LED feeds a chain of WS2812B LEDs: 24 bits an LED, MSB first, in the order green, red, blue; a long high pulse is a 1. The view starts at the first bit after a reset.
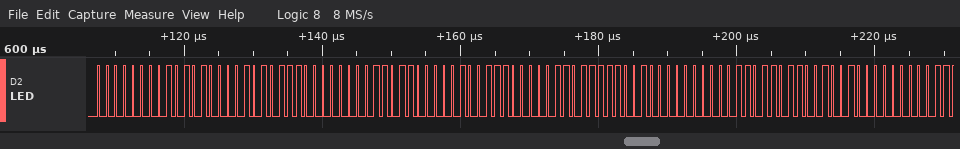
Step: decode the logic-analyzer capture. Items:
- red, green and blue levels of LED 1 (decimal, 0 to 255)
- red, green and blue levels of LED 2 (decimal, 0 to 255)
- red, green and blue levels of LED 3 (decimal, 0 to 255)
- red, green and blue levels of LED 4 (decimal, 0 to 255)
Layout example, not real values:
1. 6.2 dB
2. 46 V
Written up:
1. 168, 0, 87
2. 216, 0, 39
3. 249, 6, 0
4. 201, 54, 0
